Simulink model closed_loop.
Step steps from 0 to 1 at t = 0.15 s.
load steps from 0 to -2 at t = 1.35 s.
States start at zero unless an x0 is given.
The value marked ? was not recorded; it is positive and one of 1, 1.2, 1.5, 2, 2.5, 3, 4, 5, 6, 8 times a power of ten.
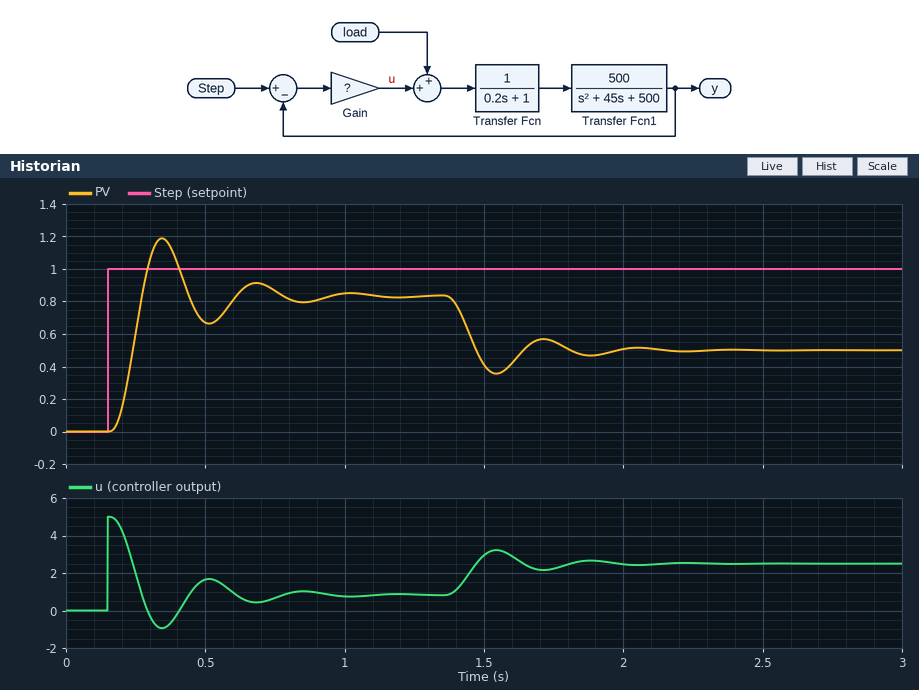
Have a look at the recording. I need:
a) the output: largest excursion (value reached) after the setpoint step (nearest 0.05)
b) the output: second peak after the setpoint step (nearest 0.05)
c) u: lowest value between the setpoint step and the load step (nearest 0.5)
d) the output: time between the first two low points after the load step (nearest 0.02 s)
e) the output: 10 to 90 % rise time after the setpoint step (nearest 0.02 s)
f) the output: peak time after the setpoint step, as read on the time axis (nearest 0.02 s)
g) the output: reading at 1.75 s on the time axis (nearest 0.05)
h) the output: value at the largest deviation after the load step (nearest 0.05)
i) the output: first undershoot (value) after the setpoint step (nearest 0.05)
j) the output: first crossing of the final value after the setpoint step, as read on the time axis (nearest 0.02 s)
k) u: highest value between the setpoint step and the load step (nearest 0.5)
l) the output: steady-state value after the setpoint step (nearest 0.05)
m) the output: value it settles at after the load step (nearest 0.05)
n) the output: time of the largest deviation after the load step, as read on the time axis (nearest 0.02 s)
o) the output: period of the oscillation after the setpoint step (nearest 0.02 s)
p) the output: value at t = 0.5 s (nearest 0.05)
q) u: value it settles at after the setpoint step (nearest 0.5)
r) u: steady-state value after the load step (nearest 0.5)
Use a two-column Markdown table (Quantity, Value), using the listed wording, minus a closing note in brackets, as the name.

| Quantity | Value |
|---|---|
| the output: largest excursion (value reached) after the setpoint step | 1.20 |
| the output: second peak after the setpoint step | 0.90 |
| u: lowest value between the setpoint step and the load step | -1.0 |
| the output: time between the first two low points after the load step | 0.34 s |
| the output: 10 to 90 % rise time after the setpoint step | 0.08 s |
| the output: peak time after the setpoint step, as read on the time axis | 0.34 s |
| the output: reading at 1.75 s on the time axis | 0.55 |
| the output: value at the largest deviation after the load step | 0.35 |
| the output: first undershoot (value) after the setpoint step | 0.65 |
| the output: first crossing of the final value after the setpoint step, as read on the time axis | 0.28 s |
| u: highest value between the setpoint step and the load step | 5.0 |
| the output: steady-state value after the setpoint step | 0.85 |
| the output: value it settles at after the load step | 0.50 |
| the output: time of the largest deviation after the load step, as read on the time axis | 1.54 s |
| the output: period of the oscillation after the setpoint step | 0.34 s |
| the output: value at t = 0.5 s | 0.65 |
| u: value it settles at after the setpoint step | 1.0 |
| u: steady-state value after the load step | 2.5 |
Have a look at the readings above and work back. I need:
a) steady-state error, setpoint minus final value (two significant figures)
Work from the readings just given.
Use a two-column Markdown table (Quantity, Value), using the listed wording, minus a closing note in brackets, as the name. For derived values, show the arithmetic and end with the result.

| Quantity | Value |
|---|---|
| steady-state error, setpoint minus final value | 1 - 0.85 = 0.15 |
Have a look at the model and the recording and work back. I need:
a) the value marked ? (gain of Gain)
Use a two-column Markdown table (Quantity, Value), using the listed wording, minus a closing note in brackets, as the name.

| Quantity | Value |
|---|---|
| the value marked ? | 5 |
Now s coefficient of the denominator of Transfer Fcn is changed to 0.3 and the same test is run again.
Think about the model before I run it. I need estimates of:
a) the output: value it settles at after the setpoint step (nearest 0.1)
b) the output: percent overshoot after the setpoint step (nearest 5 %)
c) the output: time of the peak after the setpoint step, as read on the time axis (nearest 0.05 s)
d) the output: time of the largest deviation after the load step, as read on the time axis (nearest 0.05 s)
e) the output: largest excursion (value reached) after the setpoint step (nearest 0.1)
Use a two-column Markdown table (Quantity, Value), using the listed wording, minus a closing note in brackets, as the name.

| Quantity | Value |
|---|---|
| the output: value it settles at after the setpoint step | 0.8 |
| the output: percent overshoot after the setpoint step | 30 % |
| the output: time of the peak after the setpoint step, as read on the time axis | 0.40 s |
| the output: time of the largest deviation after the load step, as read on the time axis | 1.60 s |
| the output: largest excursion (value reached) after the setpoint step | 1.1 |
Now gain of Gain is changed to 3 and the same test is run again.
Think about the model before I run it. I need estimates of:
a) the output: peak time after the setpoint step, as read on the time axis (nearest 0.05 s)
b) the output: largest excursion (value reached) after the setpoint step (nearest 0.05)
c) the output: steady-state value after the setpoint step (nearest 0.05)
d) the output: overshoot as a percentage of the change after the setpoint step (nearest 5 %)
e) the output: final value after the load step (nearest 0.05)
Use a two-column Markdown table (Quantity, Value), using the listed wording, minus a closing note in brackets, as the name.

| Quantity | Value |
|---|---|
| the output: peak time after the setpoint step, as read on the time axis | 0.40 s |
| the output: largest excursion (value reached) after the setpoint step | 0.95 |
| the output: steady-state value after the setpoint step | 0.75 |
| the output: overshoot as a percentage of the change after the setpoint step | 25 % |
| the output: final value after the load step | 0.25 |
